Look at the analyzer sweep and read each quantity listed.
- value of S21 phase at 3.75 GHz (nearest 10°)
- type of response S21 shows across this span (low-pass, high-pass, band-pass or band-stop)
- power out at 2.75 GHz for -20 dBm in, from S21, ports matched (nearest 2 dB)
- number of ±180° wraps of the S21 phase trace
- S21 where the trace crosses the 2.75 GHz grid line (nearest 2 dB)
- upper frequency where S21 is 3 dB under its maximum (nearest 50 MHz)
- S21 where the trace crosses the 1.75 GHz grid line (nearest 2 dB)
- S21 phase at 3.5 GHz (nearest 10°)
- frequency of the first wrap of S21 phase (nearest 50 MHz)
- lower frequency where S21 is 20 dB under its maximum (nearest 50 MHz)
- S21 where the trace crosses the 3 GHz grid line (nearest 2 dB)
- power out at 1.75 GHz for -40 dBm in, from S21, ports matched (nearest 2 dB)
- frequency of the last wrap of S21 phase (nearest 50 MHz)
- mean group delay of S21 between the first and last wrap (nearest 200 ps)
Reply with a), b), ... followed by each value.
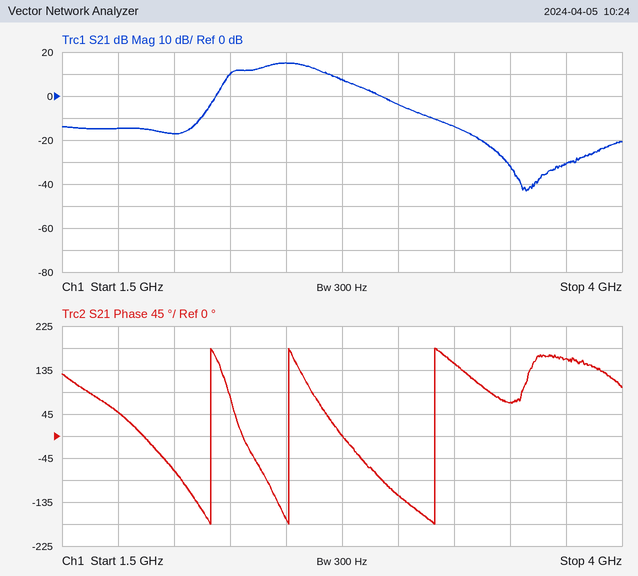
a) 160°
b) band-pass
c) -12 dBm
d) 3
e) 8 dB
f) 2.65 GHz
g) -14 dB
h) 70°
i) 2.15 GHz
j) 2.15 GHz
k) -4 dB
l) -54 dBm
m) 3.15 GHz
n) 2.0 ns
